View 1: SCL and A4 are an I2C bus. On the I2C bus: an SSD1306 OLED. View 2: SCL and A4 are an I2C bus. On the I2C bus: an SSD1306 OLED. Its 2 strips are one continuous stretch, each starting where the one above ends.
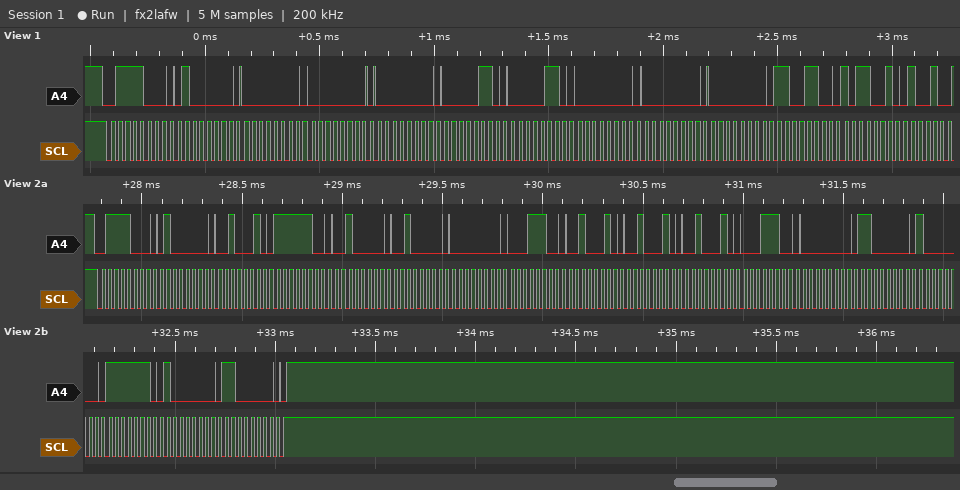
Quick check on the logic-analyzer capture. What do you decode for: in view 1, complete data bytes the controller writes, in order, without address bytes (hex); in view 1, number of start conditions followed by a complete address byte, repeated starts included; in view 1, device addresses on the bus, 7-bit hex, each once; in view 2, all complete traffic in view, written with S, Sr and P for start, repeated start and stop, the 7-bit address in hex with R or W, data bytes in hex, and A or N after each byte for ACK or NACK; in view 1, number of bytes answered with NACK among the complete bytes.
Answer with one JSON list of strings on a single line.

["40 00 00 00 06 06 00 00 00 CC B2", "1", "0x3C", "S 3CW A 40 A 22 A FC A 20 A 20 A 00 A 1C A 22 A 22 A 22 A 1C A 00 A C0 A 80 A FE A 80 A C0 A P", "0"]
